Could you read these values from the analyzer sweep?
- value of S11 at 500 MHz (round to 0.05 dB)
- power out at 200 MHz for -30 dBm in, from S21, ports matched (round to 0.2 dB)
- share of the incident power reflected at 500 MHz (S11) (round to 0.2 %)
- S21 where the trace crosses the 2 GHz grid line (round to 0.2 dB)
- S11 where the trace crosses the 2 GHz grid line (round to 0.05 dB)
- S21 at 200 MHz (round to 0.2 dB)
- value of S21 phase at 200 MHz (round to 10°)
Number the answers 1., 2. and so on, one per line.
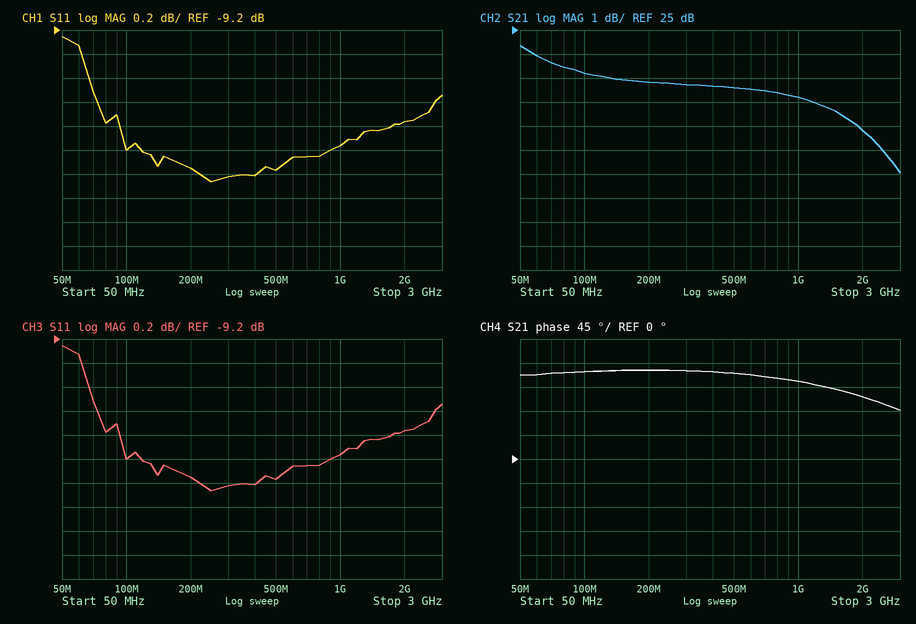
1. -10.35 dB
2. -7.2 dBm
3. 9.2 %
4. 20.8 dB
5. -9.95 dB
6. 22.8 dB
7. 170°
